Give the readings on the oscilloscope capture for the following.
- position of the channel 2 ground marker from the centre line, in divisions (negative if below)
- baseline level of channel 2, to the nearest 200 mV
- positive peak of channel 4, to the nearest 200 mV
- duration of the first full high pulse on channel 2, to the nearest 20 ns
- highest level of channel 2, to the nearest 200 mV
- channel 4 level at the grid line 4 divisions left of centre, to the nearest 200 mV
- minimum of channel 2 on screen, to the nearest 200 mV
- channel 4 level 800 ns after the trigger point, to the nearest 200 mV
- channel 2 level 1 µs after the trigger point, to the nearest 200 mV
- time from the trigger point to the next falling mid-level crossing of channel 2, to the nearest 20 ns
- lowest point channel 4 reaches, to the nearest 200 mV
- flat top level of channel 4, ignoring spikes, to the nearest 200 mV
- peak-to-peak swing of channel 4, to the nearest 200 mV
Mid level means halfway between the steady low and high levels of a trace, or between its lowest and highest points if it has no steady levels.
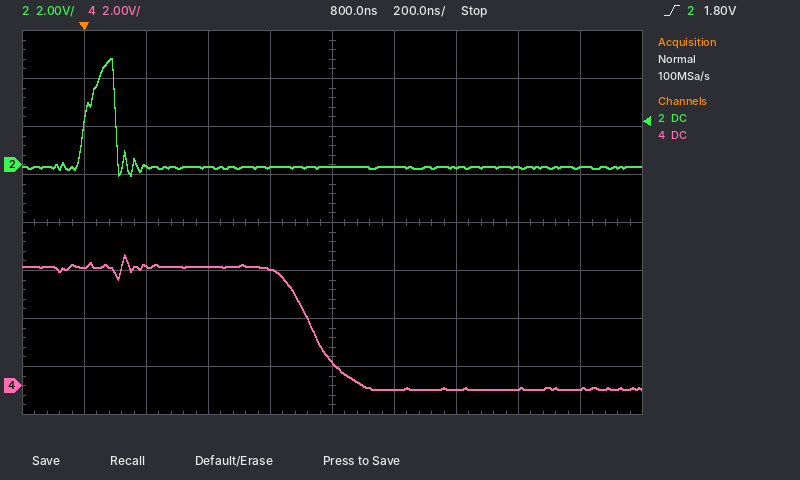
+1.2 div
0.0 V
5.4 V
100 ns
4.4 V
5.0 V
-400 mV
1.0 V
0.0 V
100 ns
-200 mV
5.0 V
5.6 V
